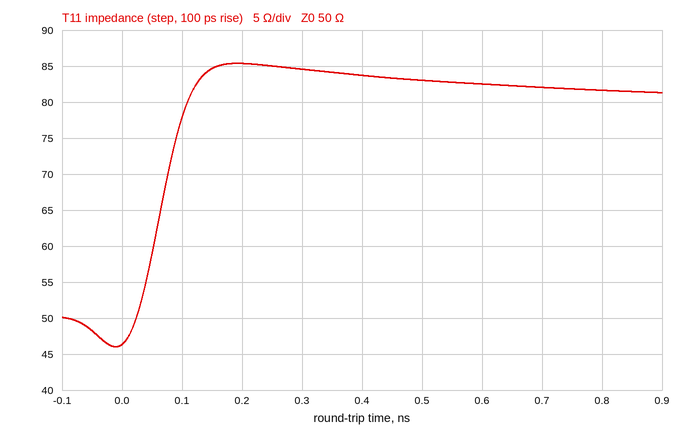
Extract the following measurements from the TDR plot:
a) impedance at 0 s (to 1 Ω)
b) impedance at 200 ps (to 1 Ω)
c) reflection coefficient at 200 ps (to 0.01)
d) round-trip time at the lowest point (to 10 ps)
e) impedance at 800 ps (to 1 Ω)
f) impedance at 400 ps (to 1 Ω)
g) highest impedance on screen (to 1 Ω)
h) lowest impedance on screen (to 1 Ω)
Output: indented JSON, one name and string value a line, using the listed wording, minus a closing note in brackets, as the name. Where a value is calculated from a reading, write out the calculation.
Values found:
{
  "impedance at 0 s": "46 Ω",
  "impedance at 200 ps": "85 Ω",
  "reflection coefficient at 200 ps": "(85 − 50)/(85 + 50) ≈ +0.26",
  "round-trip time at the lowest point": "-10 ps",
  "impedance at 800 ps": "82 Ω",
  "impedance at 400 ps": "84 Ω",
  "highest impedance on screen": "85 Ω",
  "lowest impedance on screen": "46 Ω"
}
